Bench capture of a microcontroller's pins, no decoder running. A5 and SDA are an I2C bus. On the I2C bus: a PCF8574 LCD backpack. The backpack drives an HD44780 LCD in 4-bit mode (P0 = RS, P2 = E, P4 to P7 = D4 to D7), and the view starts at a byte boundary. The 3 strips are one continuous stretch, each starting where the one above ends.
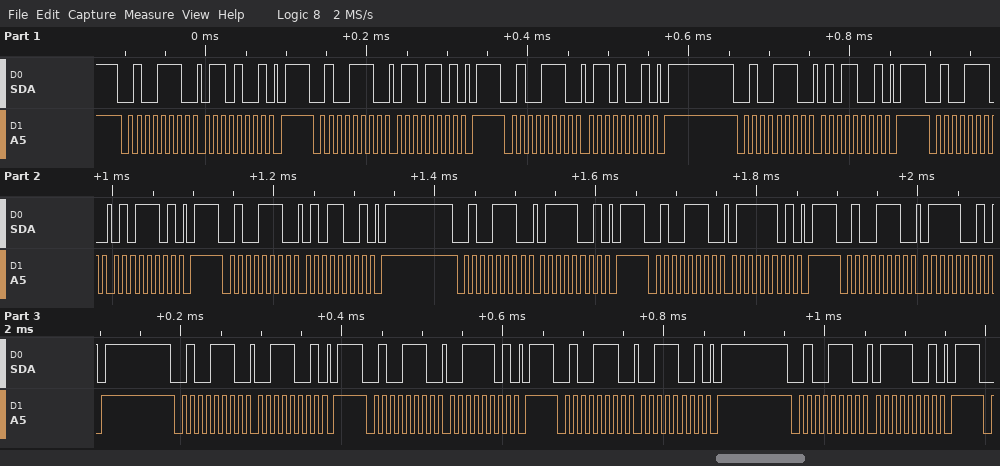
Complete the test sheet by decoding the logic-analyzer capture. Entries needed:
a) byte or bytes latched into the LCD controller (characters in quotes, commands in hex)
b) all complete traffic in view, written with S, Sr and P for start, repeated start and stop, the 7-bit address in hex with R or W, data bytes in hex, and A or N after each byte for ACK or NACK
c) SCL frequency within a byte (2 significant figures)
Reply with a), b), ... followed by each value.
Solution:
a) 'e' 's'
b) S 27W A 69 A P S 27W A 6D A P S 27W A 69 A P S 27W A 59 A P S 27W A 5D A P S 27W A 59 A P S 27W A 79 A P S 27W A 7D A P S 27W A 79 A P S 27W A 39 A P S 27W A 3D A P S 27W A 39 A P S 27W A 79 A P
c) 100 kHz
